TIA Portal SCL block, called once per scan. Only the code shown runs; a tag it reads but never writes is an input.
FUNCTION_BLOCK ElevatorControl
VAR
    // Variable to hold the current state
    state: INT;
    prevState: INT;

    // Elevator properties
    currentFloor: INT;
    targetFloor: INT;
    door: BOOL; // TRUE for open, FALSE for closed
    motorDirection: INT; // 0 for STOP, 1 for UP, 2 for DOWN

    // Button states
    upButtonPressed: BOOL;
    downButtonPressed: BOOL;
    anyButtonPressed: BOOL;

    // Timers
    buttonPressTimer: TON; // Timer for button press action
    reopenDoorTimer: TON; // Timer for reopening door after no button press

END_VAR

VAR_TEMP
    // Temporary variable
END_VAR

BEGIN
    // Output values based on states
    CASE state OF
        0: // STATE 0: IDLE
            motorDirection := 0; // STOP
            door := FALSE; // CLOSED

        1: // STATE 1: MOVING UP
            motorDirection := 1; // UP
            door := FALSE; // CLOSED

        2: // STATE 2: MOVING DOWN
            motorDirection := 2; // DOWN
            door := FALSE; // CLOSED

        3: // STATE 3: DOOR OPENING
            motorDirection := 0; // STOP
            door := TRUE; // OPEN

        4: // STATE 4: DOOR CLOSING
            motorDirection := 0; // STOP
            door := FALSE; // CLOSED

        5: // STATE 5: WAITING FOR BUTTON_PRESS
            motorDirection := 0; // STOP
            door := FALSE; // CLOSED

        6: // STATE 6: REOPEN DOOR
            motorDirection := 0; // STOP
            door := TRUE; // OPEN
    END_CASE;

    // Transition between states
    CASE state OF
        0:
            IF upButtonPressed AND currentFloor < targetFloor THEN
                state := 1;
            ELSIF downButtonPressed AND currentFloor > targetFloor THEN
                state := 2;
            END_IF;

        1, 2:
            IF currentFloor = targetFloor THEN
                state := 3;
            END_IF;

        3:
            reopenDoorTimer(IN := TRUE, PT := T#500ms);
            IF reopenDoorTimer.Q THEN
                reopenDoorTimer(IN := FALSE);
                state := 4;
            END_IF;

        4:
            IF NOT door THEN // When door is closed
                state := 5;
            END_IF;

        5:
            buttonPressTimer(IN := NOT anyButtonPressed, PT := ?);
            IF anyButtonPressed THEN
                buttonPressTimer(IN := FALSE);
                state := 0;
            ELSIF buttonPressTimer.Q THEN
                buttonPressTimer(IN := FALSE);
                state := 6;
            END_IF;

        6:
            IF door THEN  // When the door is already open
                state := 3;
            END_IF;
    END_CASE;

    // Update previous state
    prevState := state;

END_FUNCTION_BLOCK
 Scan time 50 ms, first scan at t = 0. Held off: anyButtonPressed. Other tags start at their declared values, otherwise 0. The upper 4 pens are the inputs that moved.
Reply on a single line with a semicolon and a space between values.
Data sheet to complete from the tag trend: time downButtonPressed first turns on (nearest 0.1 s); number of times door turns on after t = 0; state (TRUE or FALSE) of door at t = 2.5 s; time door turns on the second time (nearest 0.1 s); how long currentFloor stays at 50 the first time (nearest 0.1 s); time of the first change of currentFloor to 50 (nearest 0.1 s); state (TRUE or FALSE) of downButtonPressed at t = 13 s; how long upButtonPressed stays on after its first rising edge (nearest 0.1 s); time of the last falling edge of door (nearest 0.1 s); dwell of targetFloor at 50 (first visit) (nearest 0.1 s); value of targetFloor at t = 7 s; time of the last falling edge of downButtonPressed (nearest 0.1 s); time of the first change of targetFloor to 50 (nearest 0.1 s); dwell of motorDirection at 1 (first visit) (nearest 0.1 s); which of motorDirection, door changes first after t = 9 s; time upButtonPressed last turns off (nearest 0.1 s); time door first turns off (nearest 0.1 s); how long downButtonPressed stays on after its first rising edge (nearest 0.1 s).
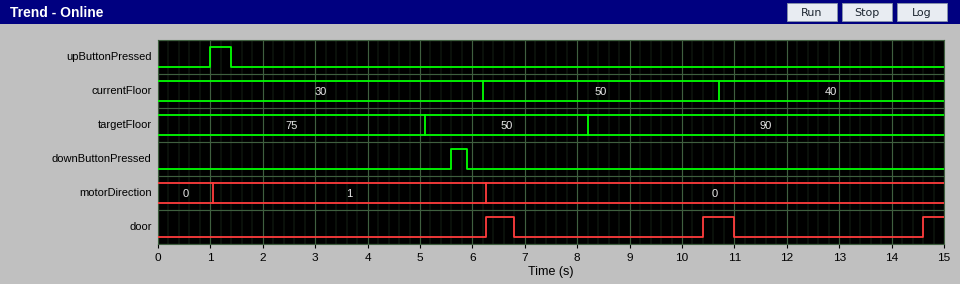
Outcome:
5.6 s; 3; FALSE; 10.4 s; 4.5 s; 6.2 s; FALSE; 0.4 s; 11.0 s; 3.1 s; 50; 5.9 s; 5.1 s; 5.2 s; door; 1.4 s; 6.8 s; 0.3 s
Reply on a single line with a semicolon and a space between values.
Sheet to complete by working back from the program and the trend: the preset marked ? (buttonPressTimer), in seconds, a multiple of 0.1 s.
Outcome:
3.5 s
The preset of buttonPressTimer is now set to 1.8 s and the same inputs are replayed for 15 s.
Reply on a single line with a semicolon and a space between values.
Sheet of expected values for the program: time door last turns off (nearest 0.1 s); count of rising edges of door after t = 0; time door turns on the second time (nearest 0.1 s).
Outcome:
14.3 s; 4; 8.7 s
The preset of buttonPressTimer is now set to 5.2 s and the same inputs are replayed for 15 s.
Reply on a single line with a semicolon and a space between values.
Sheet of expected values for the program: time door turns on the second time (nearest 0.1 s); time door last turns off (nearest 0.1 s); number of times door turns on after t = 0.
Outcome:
12.1 s; 12.7 s; 2
